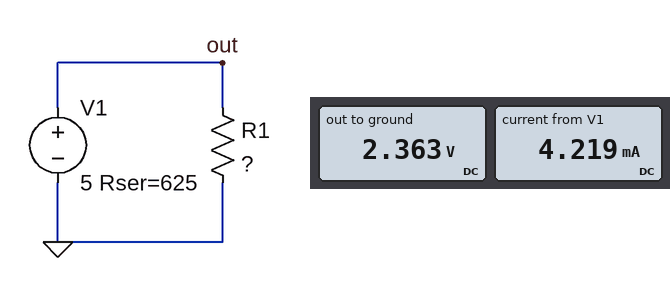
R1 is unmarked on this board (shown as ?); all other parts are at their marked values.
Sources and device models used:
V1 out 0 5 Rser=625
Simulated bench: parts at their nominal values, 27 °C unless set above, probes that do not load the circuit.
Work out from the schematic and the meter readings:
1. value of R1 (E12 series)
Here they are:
560 Ω
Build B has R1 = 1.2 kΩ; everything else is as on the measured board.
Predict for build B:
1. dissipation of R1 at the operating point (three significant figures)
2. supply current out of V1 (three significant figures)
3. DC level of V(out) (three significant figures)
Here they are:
9.01 mW
2.74 mA
3.29 V
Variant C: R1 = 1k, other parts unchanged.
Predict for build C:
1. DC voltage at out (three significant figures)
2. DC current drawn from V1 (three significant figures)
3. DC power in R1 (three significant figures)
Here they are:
3.08 V
3.08 mA
9.47 mW
